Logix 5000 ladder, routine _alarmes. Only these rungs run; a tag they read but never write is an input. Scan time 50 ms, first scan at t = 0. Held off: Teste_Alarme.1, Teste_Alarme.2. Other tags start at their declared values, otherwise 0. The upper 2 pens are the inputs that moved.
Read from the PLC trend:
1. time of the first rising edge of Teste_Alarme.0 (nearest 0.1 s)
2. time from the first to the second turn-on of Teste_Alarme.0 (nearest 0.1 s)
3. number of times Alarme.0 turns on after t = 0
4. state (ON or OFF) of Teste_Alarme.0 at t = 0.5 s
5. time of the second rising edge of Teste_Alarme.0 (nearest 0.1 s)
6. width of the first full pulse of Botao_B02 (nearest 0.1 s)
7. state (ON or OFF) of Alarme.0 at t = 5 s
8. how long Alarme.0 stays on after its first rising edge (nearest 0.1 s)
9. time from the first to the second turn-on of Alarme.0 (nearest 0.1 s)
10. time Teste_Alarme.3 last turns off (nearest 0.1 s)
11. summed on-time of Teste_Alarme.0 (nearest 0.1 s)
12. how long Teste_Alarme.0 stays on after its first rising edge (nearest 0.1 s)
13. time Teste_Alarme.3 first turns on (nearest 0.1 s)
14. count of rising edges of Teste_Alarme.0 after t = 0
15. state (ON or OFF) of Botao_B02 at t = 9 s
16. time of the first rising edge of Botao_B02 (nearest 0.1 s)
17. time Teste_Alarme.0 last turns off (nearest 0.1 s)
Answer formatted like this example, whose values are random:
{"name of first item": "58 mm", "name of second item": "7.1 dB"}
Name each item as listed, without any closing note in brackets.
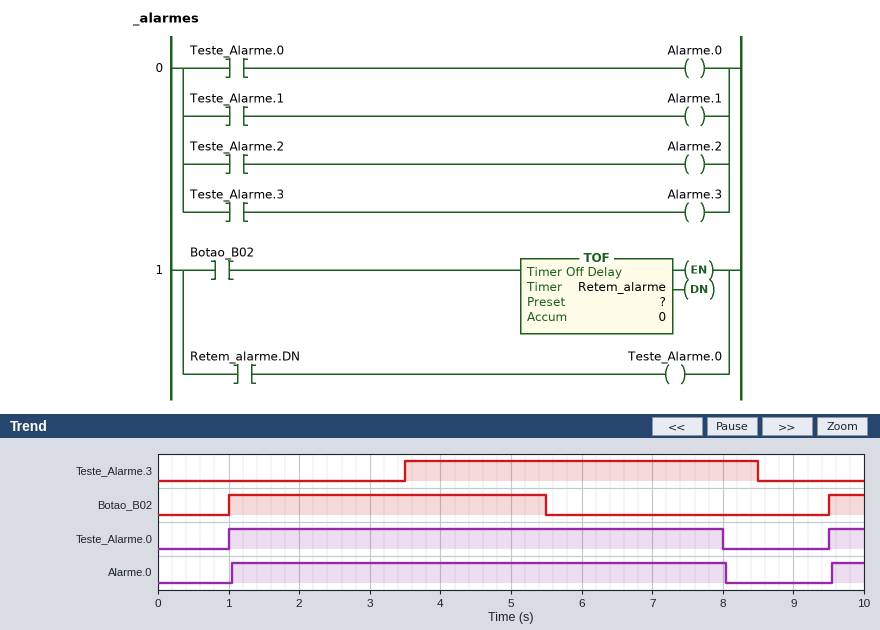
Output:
{"time of the first rising edge of Teste_Alarme.0": "1.0 s", "time from the first to the second turn-on of Teste_Alarme.0": "8.5 s", "number of times Alarme.0 turns on after t = 0": "2", "state (ON or OFF) of Teste_Alarme.0 at t = 0.5 s": "OFF", "time of the second rising edge of Teste_Alarme.0": "9.5 s", "width of the first full pulse of Botao_B02": "4.5 s", "state (ON or OFF) of Alarme.0 at t = 5 s": "ON", "how long Alarme.0 stays on after its first rising edge": "7.0 s", "time from the first to the second turn-on of Alarme.0": "8.5 s", "time Teste_Alarme.3 last turns off": "8.5 s", "summed on-time of Teste_Alarme.0": "7.5 s", "how long Teste_Alarme.0 stays on after its first rising edge": "7.0 s", "time Teste_Alarme.3 first turns on": "3.5 s", "count of rising edges of Teste_Alarme.0 after t = 0": "2", "state (ON or OFF) of Botao_B02 at t = 9 s": "OFF", "time of the first rising edge of Botao_B02": "1.0 s", "time Teste_Alarme.0 last turns off": "8.0 s"}
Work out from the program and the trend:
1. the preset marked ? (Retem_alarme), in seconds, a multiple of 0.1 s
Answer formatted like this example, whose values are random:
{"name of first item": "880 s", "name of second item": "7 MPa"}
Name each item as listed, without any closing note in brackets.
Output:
{"the preset marked ? (Retem_alarme), in seconds, a multiple of 0.1 s": "2.5 s"}
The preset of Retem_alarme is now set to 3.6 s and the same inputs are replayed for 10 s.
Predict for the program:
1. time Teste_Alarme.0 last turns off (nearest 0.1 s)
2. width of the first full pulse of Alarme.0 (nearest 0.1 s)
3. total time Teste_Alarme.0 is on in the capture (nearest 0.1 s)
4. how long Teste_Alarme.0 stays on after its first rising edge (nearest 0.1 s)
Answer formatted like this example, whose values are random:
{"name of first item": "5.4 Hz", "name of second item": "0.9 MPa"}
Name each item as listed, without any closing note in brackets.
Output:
{"time Teste_Alarme.0 last turns off": "9.1 s", "width of the first full pulse of Alarme.0": "8.1 s", "total time Teste_Alarme.0 is on in the capture": "8.6 s", "how long Teste_Alarme.0 stays on after its first rising edge": "8.1 s"}
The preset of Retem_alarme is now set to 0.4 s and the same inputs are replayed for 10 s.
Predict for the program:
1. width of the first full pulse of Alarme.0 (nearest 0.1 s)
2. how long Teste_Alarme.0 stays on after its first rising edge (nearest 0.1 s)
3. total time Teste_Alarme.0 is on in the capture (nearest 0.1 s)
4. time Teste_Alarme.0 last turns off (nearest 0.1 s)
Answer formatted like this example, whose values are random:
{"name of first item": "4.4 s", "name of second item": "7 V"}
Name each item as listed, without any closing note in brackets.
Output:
{"width of the first full pulse of Alarme.0": "4.9 s", "how long Teste_Alarme.0 stays on after its first rising edge": "4.9 s", "total time Teste_Alarme.0 is on in the capture": "5.4 s", "time Teste_Alarme.0 last turns off": "5.9 s"}
